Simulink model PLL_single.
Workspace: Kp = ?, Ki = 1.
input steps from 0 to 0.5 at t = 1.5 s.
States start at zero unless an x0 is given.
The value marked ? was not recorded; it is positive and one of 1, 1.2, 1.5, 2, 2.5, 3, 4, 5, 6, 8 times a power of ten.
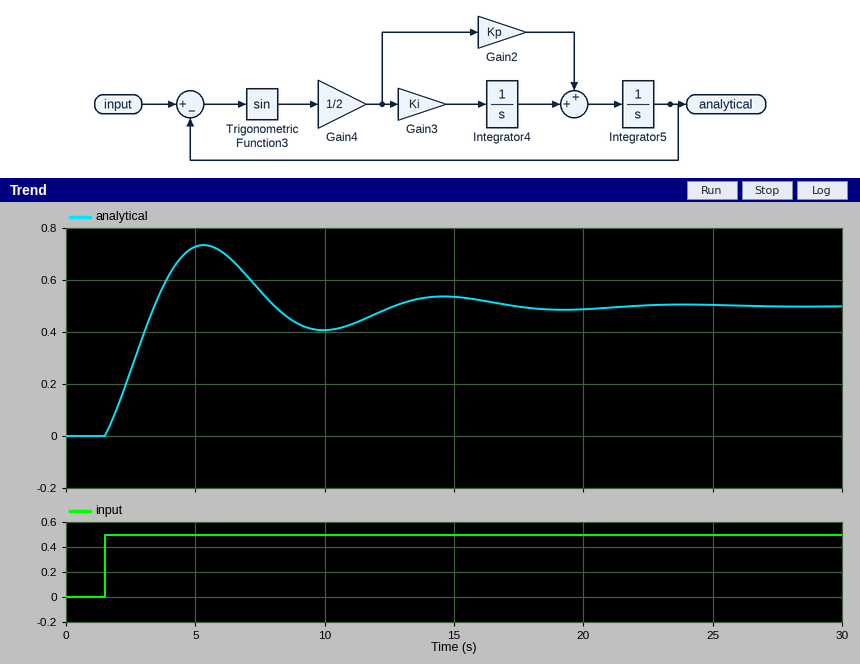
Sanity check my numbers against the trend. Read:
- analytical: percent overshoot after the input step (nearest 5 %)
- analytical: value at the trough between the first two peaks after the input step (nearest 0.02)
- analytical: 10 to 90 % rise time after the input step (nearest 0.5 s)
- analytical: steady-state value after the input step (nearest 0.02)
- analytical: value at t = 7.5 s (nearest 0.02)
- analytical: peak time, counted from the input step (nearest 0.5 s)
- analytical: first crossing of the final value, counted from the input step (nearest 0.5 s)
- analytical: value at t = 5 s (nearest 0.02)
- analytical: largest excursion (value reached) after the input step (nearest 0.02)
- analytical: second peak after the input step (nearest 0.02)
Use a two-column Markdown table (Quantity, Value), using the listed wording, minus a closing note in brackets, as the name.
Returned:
| Quantity | Value |
|---|---|
| analytical: percent overshoot after the input step | 45 % |
| analytical: value at the trough between the first two peaks after the input step | 0.40 |
| analytical: 10 to 90 % rise time after the input step | 1.5 s |
| analytical: steady-state value after the input step | 0.50 |
| analytical: value at t = 7.5 s | 0.56 |
| analytical: peak time, counted from the input step | 4.0 s |
| analytical: first crossing of the final value, counted from the input step | 2.0 s |
| analytical: value at t = 5 s | 0.72 |
| analytical: largest excursion (value reached) after the input step | 0.74 |
| analytical: second peak after the input step | 0.54 |
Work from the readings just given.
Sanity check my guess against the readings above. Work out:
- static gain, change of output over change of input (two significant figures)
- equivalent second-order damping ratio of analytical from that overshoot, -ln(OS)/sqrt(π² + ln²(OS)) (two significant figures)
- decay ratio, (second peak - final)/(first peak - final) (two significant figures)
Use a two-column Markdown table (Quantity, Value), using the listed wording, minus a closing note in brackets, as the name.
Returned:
| Quantity | Value |
|---|---|
| static gain, change of output over change of input | 1.0 |
| equivalent second-order damping ratio of analytical from that overshoot, -ln(OS)/sqrt(π² + ln²(OS)) | 0.25 |
| decay ratio, (second peak - final)/(first peak - final) | 0.17 |
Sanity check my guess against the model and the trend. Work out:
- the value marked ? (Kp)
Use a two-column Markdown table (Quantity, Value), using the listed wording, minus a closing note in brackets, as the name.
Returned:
| Quantity | Value |
|---|---|
| the value marked ? | 0.8 |
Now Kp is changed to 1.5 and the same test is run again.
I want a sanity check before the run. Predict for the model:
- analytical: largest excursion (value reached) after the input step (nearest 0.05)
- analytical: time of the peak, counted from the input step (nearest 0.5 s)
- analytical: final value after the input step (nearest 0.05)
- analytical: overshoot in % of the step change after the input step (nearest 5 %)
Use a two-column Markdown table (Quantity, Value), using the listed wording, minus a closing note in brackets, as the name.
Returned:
| Quantity | Value |
|---|---|
| analytical: largest excursion (value reached) after the input step | 0.65 |
| analytical: time of the peak, counted from the input step | 3.5 s |
| analytical: final value after the input step | 0.50 |
| analytical: overshoot in % of the step change after the input step | 30 % |
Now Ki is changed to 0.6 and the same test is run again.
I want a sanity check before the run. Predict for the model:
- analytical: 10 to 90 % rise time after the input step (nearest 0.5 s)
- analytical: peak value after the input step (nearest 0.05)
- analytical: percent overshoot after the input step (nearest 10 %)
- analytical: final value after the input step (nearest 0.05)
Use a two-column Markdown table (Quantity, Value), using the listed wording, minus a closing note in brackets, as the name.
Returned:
| Quantity | Value |
|---|---|
| analytical: 10 to 90 % rise time after the input step | 2.0 s |
| analytical: peak value after the input step | 0.70 |
| analytical: percent overshoot after the input step | 40 % |
| analytical: final value after the input step | 0.50 |
